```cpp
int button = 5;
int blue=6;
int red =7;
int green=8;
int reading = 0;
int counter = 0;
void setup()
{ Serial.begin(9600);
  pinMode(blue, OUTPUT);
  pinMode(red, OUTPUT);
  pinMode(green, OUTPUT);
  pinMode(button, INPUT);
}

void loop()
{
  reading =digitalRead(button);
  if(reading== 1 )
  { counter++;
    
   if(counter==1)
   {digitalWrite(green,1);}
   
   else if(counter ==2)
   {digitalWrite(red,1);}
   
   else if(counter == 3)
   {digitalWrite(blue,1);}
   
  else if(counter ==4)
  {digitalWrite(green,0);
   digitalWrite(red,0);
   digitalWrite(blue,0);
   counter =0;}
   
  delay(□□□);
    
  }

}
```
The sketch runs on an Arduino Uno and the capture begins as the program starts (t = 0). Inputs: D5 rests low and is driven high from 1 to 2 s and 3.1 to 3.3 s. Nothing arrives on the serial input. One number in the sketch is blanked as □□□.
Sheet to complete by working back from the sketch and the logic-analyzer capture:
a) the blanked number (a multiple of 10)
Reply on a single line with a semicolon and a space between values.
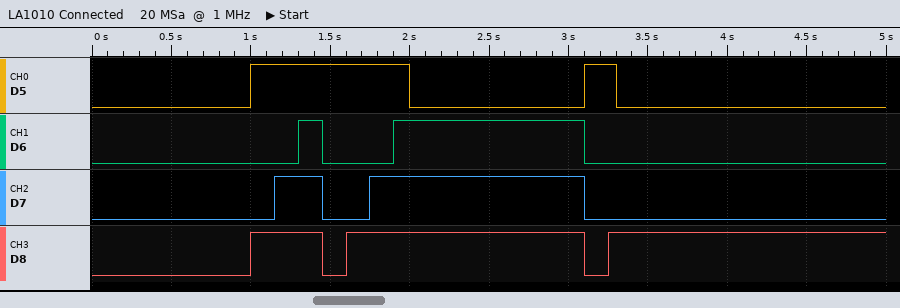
150
